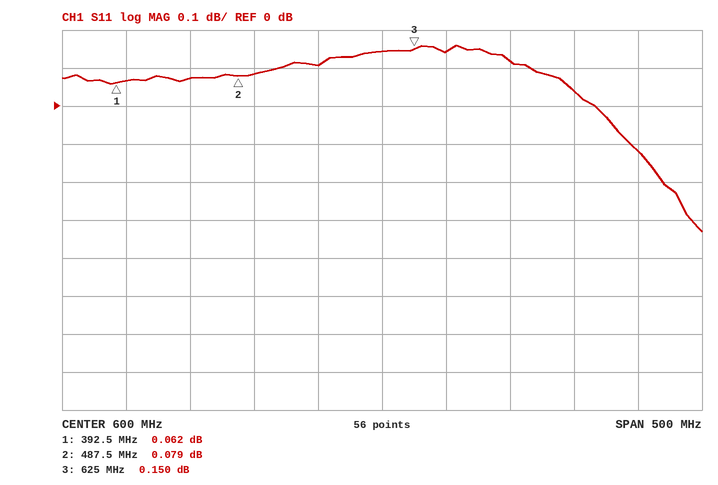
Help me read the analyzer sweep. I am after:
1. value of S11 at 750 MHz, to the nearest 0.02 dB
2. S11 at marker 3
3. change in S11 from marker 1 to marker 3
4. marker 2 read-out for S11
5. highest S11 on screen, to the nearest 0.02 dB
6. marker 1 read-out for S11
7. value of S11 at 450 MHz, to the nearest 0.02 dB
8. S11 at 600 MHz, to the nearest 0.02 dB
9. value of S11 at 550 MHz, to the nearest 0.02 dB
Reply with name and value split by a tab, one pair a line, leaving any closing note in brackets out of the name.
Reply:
value of S11 at 750 MHz, to the nearest 0.02 dB	0.04 dB
S11 at marker 3	0.150 dB
change in S11 from marker 1 to marker 3	0.088 dB
marker 2 read-out for S11	0.079 dB
highest S11 on screen, to the nearest 0.02 dB	0.16 dB
marker 1 read-out for S11	0.062 dB
value of S11 at 450 MHz, to the nearest 0.02 dB	0.08 dB
S11 at 600 MHz, to the nearest 0.02 dB	0.14 dB
value of S11 at 550 MHz, to the nearest 0.02 dB	0.10 dB
